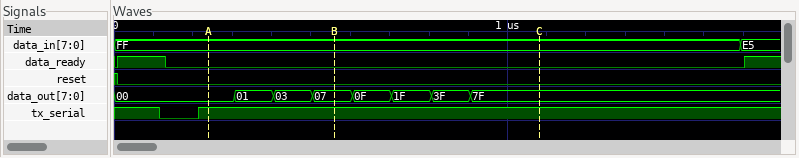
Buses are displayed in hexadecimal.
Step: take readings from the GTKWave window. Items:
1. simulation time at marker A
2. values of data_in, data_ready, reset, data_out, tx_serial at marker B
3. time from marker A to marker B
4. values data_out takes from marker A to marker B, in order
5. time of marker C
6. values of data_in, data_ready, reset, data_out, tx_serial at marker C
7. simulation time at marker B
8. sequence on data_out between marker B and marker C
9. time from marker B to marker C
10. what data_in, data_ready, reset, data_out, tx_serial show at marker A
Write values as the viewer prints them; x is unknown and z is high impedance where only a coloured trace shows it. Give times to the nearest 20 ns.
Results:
240 ns
data_in=FF, data_ready=0, reset=0, data_out=07, tx_serial=1
320 ns
00, 01, 03, 07
1080 ns
data_in=FF, data_ready=0, reset=0, data_out=7F, tx_serial=1
560 ns
07, 0F, 1F, 3F, 7F
520 ns
data_in=FF, data_ready=0, reset=0, data_out=00, tx_serial=1
